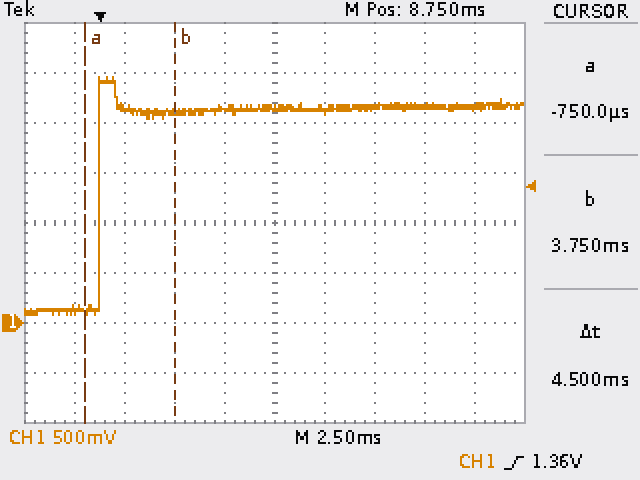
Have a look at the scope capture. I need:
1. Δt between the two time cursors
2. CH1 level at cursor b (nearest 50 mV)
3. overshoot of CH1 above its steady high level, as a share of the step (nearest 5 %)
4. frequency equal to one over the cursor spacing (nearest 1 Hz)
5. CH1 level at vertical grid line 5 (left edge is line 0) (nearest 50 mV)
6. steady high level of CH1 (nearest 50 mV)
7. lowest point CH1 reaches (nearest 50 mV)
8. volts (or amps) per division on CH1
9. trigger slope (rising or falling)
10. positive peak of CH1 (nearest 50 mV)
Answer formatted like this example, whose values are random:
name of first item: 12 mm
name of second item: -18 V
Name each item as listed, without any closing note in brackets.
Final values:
Δt between the two time cursors: 4.5 ms
CH1 level at cursor b: 2.10 V
overshoot of CH1 above its steady high level, as a share of the step: 15 %
frequency equal to one over the cursor spacing: 222 Hz
CH1 level at vertical grid line 5 (left edge is line 0): 2.15 V
steady high level of CH1: 2.15 V
lowest point CH1 reaches: 100 mV
volts (or amps) per division on CH1: 500 mV
trigger slope: rising
positive peak of CH1: 2.45 V
